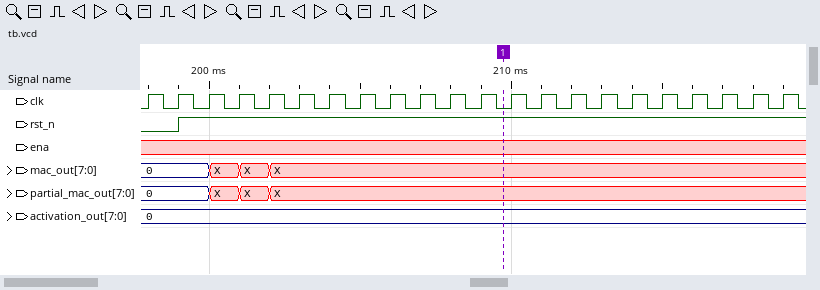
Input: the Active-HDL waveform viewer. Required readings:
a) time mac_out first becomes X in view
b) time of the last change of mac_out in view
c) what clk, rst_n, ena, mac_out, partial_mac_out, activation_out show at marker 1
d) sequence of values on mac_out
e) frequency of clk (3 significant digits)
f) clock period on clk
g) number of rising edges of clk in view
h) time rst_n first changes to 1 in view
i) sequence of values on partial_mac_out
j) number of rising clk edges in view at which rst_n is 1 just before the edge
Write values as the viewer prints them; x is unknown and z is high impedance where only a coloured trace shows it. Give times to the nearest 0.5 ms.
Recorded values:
200 ms
202 ms
clk=0, rst_n=1, ena=x, mac_out=X, partial_mac_out=X, activation_out=0
0, X, X, X
1.00 kHz
1 ms
22
199 ms
0, X, X, X
20
